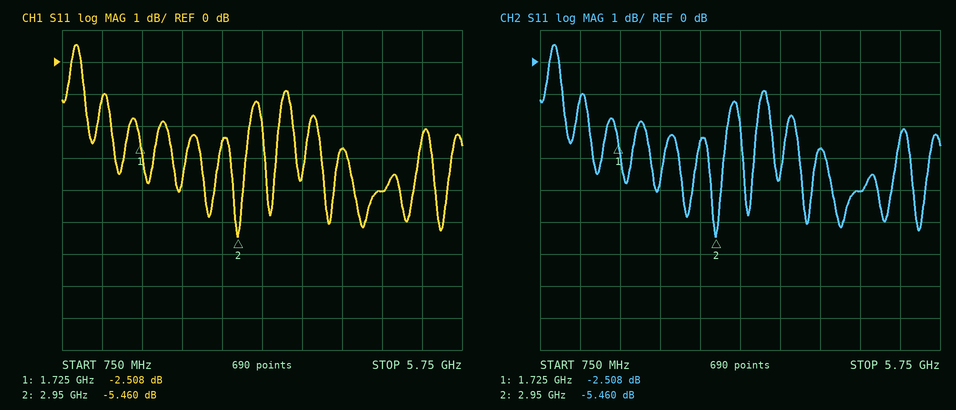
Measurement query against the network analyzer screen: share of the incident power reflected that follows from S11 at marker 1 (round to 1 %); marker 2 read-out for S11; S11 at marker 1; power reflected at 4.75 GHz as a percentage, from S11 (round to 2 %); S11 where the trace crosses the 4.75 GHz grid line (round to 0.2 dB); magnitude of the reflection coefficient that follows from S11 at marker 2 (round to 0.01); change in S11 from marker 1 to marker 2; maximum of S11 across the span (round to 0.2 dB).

56 %
-5.460 dB
-2.508 dB
40 %
-4.0 dB
0.53
-2.952 dB
0.6 dB
